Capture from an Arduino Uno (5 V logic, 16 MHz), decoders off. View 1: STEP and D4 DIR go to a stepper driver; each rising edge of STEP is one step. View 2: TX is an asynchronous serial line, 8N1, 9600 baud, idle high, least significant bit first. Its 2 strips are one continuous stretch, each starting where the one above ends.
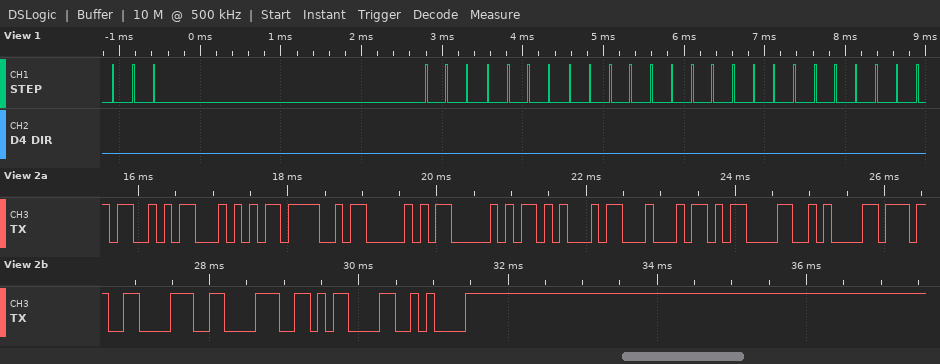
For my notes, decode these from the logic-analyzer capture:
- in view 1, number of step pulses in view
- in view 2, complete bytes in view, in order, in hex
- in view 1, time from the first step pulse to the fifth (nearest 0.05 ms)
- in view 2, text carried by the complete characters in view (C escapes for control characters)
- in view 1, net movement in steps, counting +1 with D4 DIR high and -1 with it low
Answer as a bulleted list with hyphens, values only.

- 28
- 53 54 4F 50 50 45 44 0D 0A 37 38 38 0D 0A
- 4.15 ms
- "STOPPED\r\n788\r\n"
- -28
